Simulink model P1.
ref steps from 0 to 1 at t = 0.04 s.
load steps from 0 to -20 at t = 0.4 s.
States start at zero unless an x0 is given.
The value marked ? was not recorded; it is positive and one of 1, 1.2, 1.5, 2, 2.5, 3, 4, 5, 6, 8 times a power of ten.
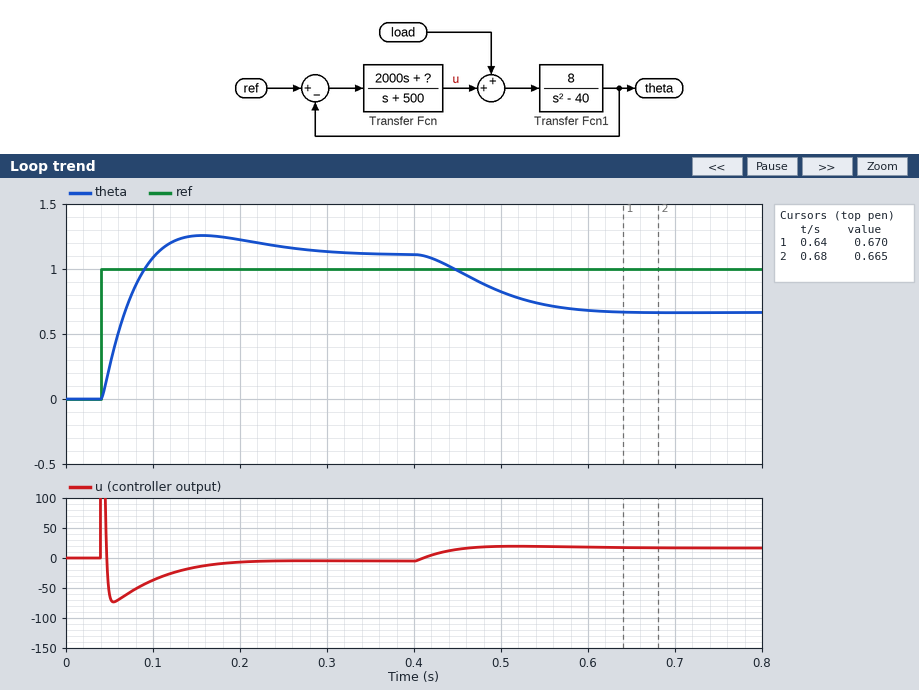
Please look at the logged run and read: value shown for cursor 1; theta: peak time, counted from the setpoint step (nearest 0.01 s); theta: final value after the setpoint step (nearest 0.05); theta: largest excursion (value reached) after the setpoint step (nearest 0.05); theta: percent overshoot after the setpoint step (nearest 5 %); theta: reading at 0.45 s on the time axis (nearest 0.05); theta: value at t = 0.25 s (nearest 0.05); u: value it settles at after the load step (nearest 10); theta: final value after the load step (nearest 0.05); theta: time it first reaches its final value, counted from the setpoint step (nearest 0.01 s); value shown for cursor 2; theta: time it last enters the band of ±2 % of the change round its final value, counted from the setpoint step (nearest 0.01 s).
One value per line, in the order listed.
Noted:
0.670
0.12 s
1.10
1.25
15 %
1.00
1.15
20
0.65
0.06 s
0.665
0.26 s
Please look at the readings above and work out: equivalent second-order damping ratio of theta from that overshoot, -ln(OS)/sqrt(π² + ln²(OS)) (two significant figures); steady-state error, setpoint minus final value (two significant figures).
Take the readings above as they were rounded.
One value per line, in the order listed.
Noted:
0.52
-0.10
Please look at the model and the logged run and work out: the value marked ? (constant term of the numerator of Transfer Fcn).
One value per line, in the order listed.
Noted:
25000
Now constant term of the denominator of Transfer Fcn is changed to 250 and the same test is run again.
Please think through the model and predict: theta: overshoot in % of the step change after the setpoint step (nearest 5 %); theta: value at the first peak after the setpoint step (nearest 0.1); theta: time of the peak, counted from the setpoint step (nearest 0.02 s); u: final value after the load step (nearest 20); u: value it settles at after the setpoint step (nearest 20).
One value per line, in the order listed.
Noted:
10 %
1.2
0.06 s
20
0
